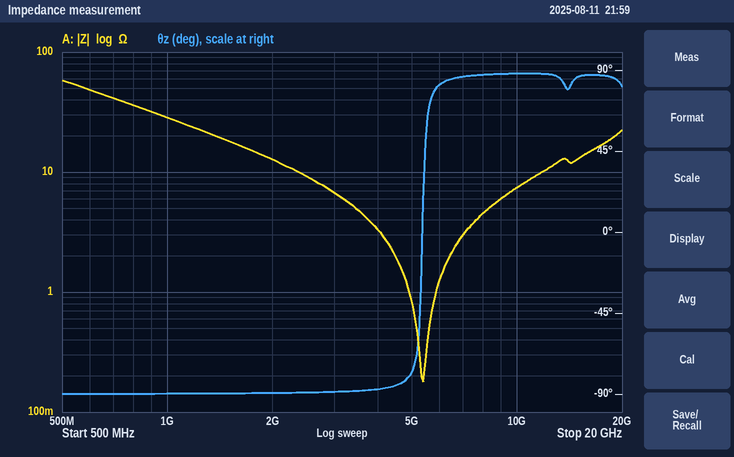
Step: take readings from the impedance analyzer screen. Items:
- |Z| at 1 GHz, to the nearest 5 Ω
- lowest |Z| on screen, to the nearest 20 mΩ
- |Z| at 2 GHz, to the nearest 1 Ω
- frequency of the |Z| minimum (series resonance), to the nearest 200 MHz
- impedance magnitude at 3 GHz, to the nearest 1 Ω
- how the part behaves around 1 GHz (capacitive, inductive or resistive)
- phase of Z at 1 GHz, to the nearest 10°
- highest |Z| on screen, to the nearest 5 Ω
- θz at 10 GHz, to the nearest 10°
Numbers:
30 Ω
180 mΩ
13 Ω
5.4 GHz
7 Ω
capacitive
-90°
60 Ω
90°
